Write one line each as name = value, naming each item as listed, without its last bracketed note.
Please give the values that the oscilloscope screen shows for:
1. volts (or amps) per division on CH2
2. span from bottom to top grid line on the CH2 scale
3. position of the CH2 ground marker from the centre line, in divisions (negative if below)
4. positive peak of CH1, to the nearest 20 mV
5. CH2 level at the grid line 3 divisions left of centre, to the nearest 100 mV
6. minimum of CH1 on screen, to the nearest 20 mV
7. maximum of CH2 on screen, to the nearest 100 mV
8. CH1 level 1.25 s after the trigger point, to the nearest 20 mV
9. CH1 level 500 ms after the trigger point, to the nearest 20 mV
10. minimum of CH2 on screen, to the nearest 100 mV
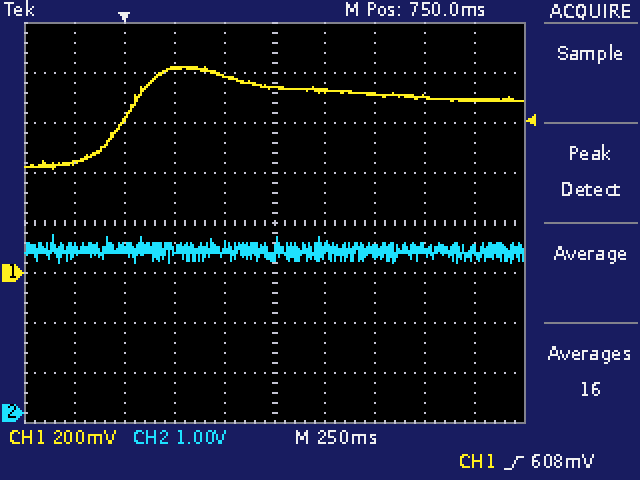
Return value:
volts (or amps) per division on CH2 = 1 V
span from bottom to top grid line on the CH2 scale = 8 V
position of the CH2 ground marker from the centre line, in divisions = -3.8 div
positive peak of CH1, to the nearest 20 mV = 820 mV
CH2 level at the grid line 3 divisions left of centre, to the nearest 100 mV = 3.3 V
minimum of CH1 on screen, to the nearest 20 mV = 420 mV
maximum of CH2 on screen, to the nearest 100 mV = 3.6 V
CH1 level 1.25 s after the trigger point, to the nearest 20 mV = 720 mV
CH1 level 500 ms after the trigger point, to the nearest 20 mV = 780 mV
minimum of CH2 on screen, to the nearest 100 mV = 3.0 V
